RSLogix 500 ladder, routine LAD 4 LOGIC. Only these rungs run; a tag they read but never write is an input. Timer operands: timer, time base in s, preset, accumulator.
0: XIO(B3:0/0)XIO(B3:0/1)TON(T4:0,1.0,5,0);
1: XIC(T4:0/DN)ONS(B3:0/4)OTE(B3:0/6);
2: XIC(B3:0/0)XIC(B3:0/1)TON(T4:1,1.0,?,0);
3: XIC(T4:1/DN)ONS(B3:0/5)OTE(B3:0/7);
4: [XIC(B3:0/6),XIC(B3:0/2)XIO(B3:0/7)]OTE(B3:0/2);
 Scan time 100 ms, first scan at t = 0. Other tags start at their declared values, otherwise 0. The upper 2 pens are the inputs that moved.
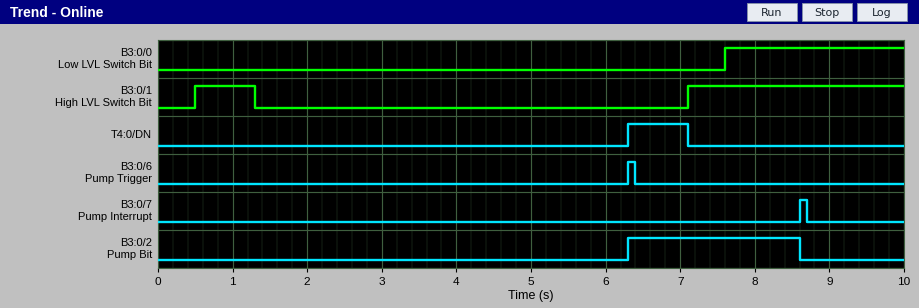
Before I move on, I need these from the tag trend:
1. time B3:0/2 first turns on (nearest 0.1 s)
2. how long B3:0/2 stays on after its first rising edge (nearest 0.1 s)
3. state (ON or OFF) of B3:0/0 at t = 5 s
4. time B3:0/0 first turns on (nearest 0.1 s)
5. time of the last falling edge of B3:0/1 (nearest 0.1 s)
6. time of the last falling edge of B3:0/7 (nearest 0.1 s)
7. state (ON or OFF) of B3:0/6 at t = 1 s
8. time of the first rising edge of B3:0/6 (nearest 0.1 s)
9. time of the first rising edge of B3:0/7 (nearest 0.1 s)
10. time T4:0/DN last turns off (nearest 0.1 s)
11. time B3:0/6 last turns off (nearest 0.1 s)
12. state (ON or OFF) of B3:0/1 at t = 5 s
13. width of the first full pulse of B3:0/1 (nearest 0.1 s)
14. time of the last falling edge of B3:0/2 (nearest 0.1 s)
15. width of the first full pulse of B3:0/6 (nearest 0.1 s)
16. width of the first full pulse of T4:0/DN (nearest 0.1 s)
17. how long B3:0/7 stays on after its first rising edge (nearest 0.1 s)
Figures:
6.3 s
2.3 s
OFF
7.6 s
1.3 s
8.7 s
OFF
6.3 s
8.6 s
7.1 s
6.4 s
OFF
0.8 s
8.6 s
0.1 s
0.8 s
0.1 s
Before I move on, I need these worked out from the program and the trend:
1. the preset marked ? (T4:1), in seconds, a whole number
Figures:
1 s
